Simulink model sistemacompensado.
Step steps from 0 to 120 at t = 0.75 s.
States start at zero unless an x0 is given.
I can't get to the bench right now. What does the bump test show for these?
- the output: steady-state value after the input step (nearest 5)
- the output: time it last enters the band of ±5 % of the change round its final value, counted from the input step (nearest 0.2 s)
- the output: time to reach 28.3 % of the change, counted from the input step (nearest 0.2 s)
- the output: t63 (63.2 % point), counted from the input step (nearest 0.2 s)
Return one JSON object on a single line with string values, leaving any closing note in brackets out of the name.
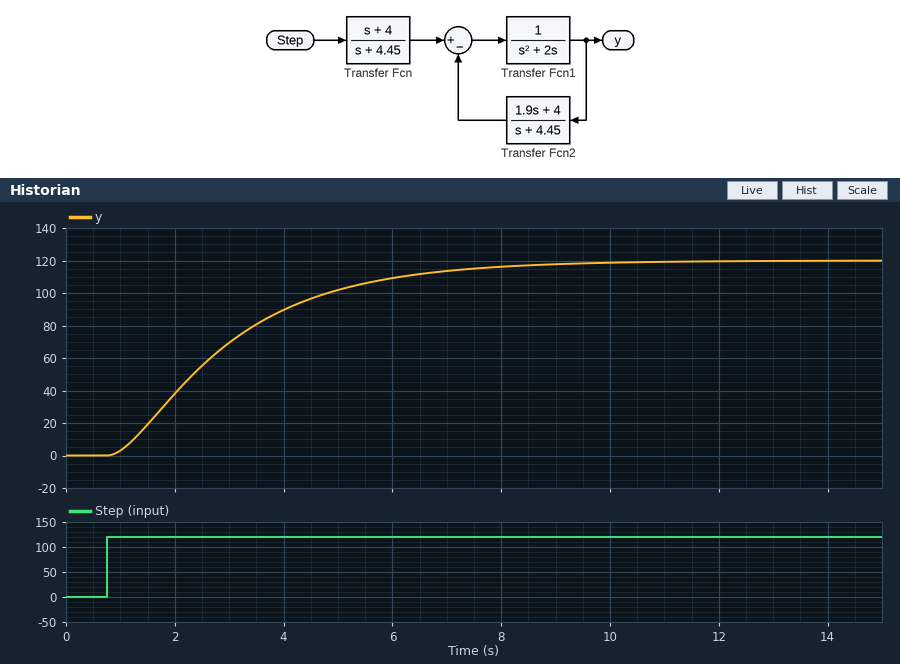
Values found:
{"the output: steady-state value after the input step": "120", "the output: time it last enters the band of ±5 % of the change round its final value, counted from the input step": "6.4 s", "the output: time to reach 28.3 % of the change, counted from the input step": "1.2 s", "the output: t63 (63.2 % point), counted from the input step": "2.6 s"}
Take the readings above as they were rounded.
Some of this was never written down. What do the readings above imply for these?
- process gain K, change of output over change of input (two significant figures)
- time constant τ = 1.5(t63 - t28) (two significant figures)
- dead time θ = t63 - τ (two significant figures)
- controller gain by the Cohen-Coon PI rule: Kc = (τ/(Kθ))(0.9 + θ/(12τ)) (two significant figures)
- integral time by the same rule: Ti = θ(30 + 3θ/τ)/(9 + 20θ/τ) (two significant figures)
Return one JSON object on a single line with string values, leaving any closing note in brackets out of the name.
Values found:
{"process gain K, change of output over change of input": "1.0", "time constant τ = 1.5(t63 - t28)": "2.1 s", "dead time θ = t63 - τ": "0.50 s", "controller gain by the Cohen-Coon PI rule: Kc = (τ/(Kθ))(0.9 + θ/(12τ))": "3.9", "integral time by the same rule: Ti = θ(30 + 3θ/τ)/(9 + 20θ/τ)": "1.1 s"}
